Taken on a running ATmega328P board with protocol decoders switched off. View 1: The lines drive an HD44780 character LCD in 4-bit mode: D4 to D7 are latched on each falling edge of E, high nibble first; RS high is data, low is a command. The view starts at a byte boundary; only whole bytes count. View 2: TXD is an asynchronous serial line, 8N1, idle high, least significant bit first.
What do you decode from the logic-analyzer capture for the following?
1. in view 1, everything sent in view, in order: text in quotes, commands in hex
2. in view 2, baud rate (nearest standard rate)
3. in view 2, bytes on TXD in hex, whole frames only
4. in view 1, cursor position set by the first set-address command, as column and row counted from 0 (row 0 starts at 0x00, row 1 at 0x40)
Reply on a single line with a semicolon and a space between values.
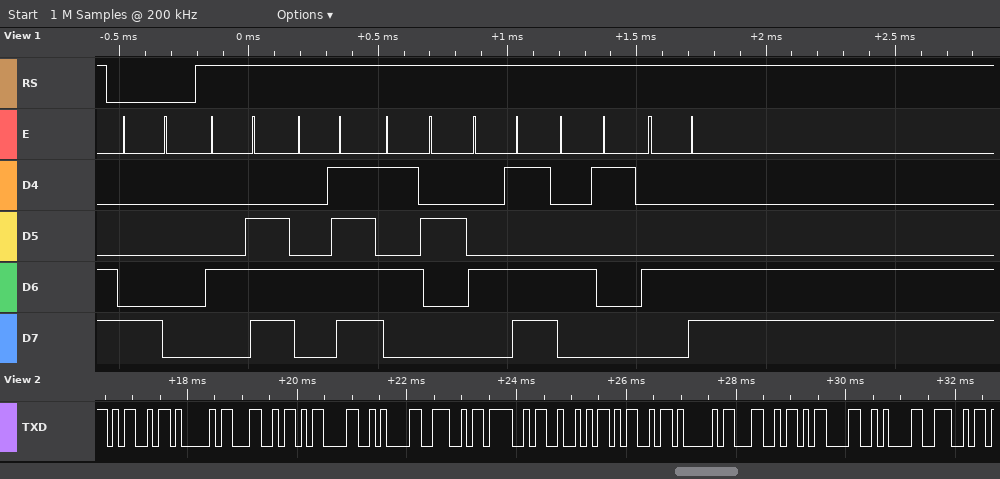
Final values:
0x80 "NORMAL"; 9600 baud; 0x4D 0x41 0x4C 0x0D 0x0A 0x4E 0x4F 0x52 0x4D 0x41 0x4C 0x0D 0x0A 0x4E; column 0, row 0
